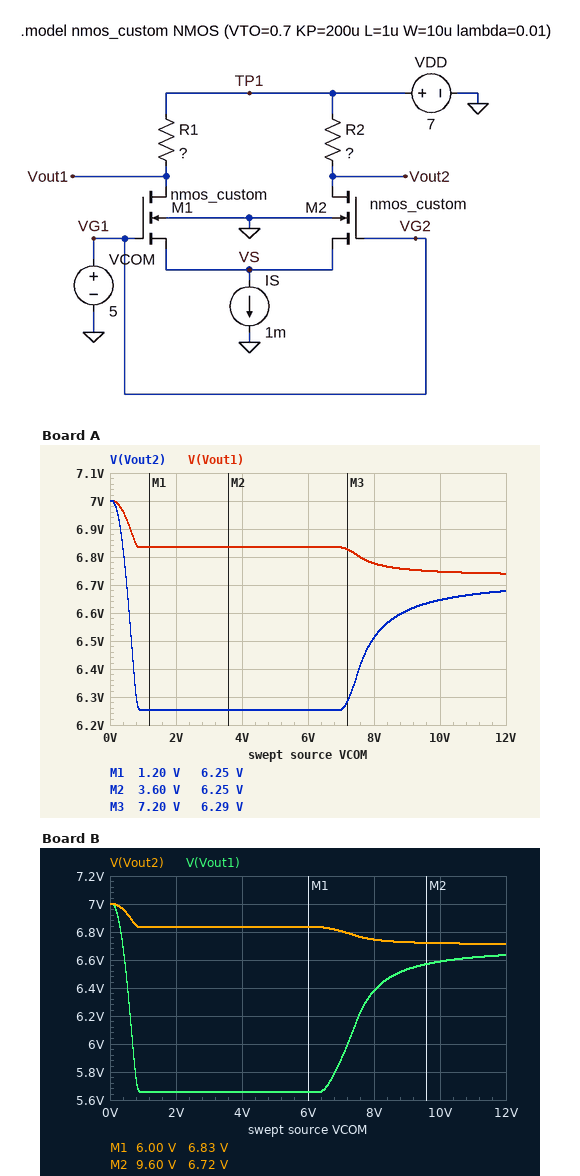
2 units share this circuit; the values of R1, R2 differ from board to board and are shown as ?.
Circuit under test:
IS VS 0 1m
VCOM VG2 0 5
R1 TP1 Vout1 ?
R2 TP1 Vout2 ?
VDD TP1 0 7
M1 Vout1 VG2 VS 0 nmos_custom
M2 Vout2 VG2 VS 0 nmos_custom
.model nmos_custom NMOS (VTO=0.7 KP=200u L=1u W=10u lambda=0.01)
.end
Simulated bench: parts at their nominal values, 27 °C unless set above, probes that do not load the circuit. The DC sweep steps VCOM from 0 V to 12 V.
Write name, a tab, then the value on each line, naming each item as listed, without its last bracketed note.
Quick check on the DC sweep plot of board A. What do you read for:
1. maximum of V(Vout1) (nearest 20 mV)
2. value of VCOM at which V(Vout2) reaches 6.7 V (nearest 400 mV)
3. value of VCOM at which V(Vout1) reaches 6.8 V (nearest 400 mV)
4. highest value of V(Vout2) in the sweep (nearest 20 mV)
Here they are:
maximum of V(Vout1)	7.00 V
value of VCOM at which V(Vout2) reaches 6.7 V	400 mV
value of VCOM at which V(Vout1) reaches 6.8 V	7.6 V
highest value of V(Vout2) in the sweep	7.00 V
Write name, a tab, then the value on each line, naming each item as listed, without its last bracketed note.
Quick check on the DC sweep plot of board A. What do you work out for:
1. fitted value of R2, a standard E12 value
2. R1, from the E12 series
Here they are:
fitted value of R2, a standard E12 value	1.5 kΩ
R1, from the E12 series	330 Ω
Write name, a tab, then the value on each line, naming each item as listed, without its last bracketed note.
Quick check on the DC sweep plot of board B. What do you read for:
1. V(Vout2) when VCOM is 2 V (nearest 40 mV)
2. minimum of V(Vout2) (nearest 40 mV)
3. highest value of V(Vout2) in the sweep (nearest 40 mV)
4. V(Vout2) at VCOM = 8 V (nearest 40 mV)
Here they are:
V(Vout2) when VCOM is 2 V	6.84 V
minimum of V(Vout2)	6.72 V
highest value of V(Vout2) in the sweep	7.00 V
V(Vout2) at VCOM = 8 V	6.76 V
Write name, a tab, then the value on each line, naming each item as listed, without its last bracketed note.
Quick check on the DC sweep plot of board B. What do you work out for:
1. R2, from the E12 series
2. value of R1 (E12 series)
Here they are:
R2, from the E12 series	330 Ω
value of R1	2.7 kΩ
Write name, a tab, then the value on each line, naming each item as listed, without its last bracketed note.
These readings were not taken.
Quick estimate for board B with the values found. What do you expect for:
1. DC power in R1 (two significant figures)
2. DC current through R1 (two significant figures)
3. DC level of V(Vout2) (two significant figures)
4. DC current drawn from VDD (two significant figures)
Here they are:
DC power in R1	670 µW
DC current through R1	500 µA
DC level of V(Vout2)	6.8 V
DC current drawn from VDD	1.0 mA
